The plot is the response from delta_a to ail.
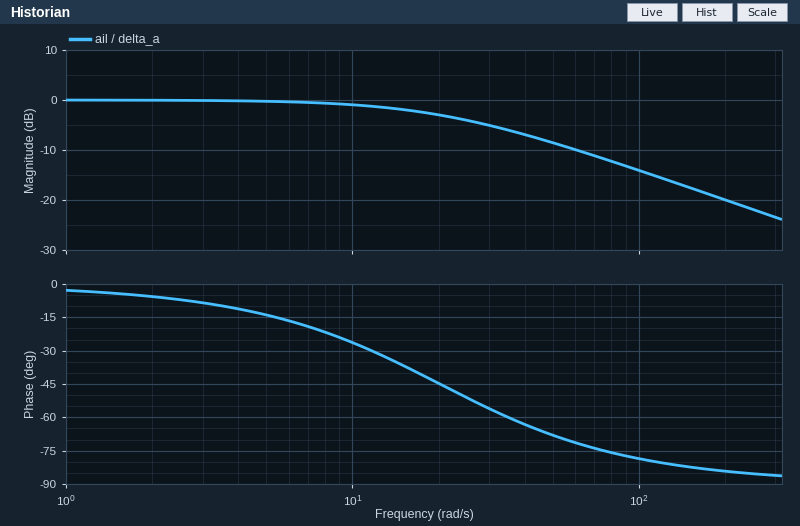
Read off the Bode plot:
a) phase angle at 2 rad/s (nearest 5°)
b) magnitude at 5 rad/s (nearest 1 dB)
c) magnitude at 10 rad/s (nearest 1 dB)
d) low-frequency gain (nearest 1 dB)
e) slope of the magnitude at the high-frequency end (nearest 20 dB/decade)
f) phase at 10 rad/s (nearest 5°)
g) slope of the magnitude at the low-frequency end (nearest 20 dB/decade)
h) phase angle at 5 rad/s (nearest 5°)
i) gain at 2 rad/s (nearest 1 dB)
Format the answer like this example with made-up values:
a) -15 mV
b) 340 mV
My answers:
a) -5°
b) 0 dB
c) -1 dB
d) 0 dB
e) -20 dB/decade
f) -25°
g) 0 dB/decade
h) -15°
i) 0 dB
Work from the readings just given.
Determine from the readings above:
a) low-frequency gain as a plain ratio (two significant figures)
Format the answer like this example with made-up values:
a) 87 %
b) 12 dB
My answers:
a) 1.0
